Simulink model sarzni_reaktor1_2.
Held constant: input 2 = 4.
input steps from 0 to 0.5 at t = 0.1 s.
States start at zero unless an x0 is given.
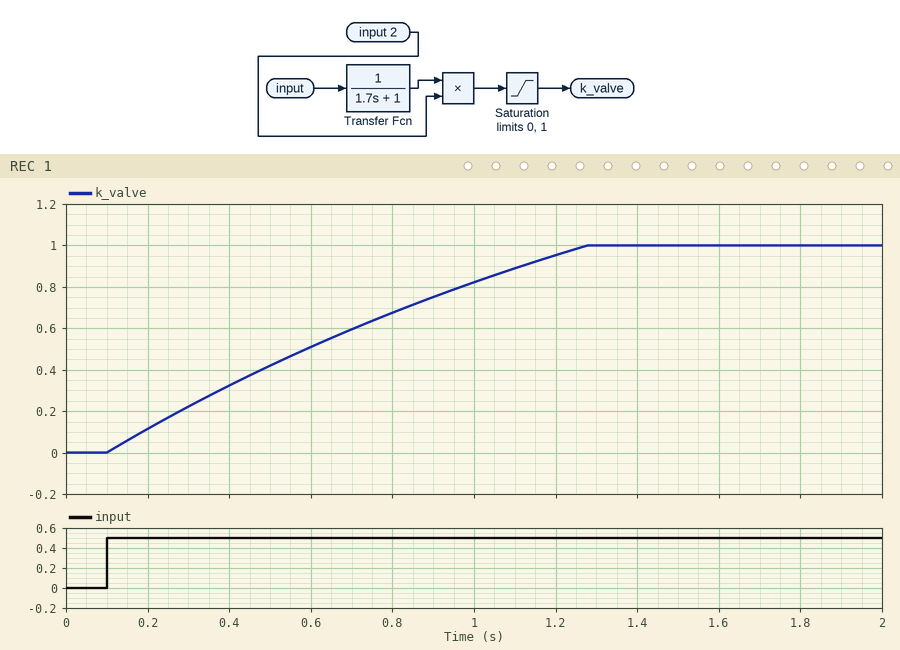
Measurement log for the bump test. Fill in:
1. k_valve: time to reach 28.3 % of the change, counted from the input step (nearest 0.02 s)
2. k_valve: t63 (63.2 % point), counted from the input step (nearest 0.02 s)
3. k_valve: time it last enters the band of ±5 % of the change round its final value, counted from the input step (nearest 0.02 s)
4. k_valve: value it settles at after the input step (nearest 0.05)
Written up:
0.26 s
0.64 s
1.10 s
1.00
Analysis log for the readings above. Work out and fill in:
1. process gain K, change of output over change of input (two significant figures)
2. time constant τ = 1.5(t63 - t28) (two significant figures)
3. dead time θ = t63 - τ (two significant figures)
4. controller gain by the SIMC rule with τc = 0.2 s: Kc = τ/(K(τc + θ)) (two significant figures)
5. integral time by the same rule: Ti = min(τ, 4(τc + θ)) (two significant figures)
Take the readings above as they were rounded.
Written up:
2.0
0.57 s
0.070 s
1.1
0.57 s
